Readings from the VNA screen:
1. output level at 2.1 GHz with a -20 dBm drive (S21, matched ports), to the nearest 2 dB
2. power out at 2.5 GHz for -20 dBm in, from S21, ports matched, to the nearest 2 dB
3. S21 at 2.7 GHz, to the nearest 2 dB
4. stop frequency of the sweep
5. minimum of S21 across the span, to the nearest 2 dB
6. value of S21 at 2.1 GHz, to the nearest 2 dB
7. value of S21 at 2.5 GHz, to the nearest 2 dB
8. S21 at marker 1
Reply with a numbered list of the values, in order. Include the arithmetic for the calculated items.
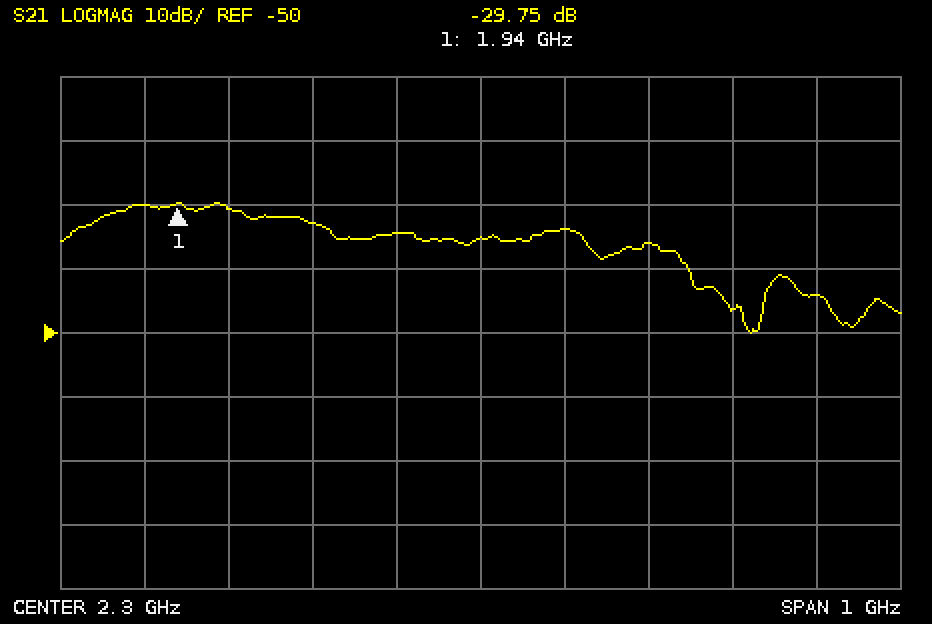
1. -20 dBm + (-32 dB) = -52 dBm
2. -20 dBm + (-36 dB) = -56 dBm
3. -44 dB
4. 2.8 GHz
5. -50 dB
6. -32 dB
7. -36 dB
8. -29.75 dB
